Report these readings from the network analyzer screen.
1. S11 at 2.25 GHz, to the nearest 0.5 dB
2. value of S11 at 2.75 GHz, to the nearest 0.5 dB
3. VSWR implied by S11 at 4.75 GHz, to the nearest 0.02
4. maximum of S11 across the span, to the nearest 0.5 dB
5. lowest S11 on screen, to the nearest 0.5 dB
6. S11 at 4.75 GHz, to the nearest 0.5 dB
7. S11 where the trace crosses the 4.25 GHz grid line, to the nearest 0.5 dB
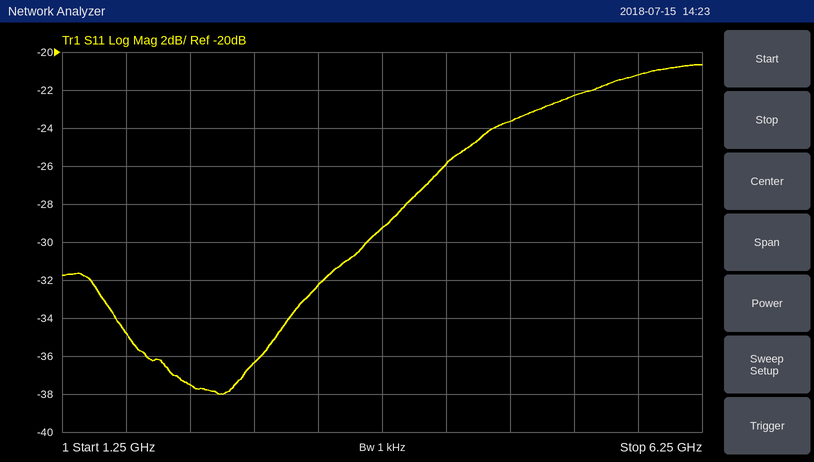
-37.5 dB
-36.5 dB
1.14
-20.5 dB
-38.0 dB
-23.5 dB
-26.0 dB
